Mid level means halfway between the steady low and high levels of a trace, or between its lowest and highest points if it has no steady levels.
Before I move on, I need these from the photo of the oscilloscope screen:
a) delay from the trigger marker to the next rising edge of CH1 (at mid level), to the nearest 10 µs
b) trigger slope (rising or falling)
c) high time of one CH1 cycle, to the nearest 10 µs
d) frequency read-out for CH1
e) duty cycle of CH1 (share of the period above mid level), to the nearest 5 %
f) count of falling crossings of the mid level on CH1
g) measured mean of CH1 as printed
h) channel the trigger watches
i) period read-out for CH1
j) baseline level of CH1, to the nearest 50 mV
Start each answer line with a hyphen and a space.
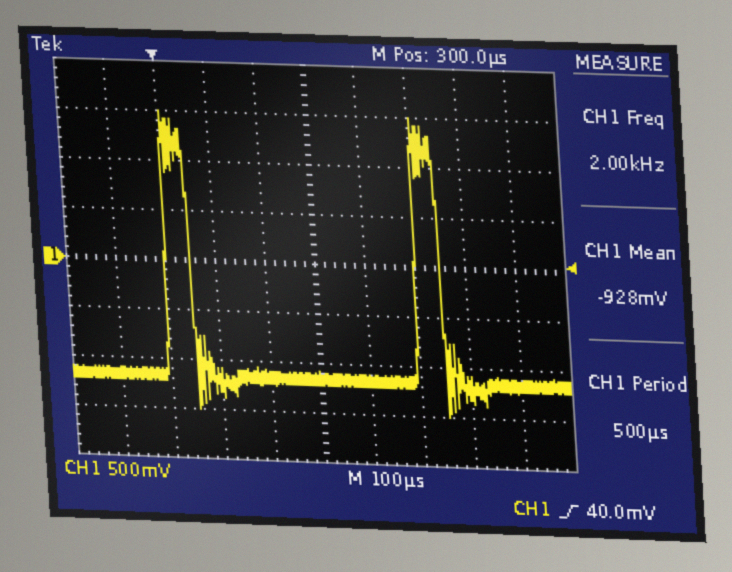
- 500 µs
- rising
- 50 µs
- 2.00 kHz
- 10 %
- 2
- -928 mV
- CH1
- 500 µs
- -1.15 V
